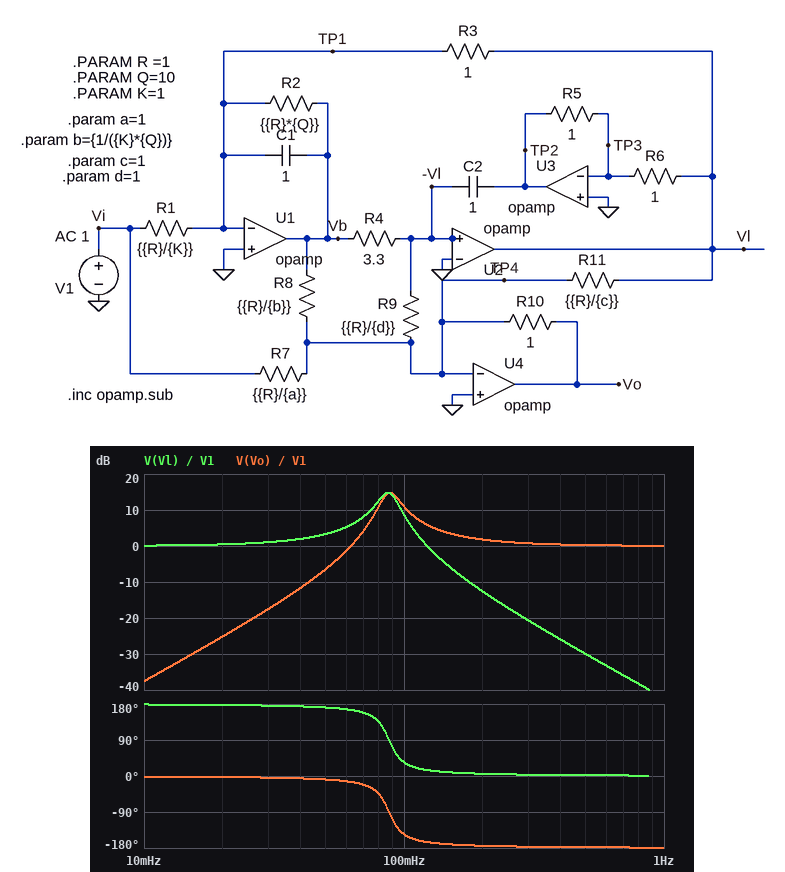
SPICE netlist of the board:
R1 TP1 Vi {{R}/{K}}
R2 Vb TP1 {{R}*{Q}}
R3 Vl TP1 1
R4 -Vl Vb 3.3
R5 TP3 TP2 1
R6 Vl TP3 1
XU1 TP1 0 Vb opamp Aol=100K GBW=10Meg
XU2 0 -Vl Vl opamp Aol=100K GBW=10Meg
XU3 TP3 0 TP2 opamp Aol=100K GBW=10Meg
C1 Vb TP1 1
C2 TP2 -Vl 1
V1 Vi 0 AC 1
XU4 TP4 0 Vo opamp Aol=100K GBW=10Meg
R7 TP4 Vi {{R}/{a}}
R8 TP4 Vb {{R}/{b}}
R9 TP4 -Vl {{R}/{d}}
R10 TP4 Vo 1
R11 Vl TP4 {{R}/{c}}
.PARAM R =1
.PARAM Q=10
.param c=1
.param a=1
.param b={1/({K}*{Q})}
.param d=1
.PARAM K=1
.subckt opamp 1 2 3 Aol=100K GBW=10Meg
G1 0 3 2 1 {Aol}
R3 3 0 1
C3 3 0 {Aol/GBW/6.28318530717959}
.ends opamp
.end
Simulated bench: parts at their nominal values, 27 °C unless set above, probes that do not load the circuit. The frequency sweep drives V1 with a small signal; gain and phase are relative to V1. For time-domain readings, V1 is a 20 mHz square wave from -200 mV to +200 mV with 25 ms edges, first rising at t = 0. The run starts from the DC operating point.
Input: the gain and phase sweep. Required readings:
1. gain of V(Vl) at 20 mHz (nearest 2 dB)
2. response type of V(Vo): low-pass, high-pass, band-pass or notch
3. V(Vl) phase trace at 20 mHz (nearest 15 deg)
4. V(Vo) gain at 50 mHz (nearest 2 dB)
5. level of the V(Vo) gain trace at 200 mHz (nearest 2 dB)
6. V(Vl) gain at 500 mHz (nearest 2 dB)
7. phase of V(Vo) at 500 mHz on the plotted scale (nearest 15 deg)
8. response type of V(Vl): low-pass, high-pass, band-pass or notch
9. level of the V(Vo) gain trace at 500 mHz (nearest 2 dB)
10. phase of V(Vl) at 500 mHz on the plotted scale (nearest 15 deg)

0 dB
high-pass
180 deg
-6 dB
2 dB
-30 dB
-180 deg
low-pass
0 dB
0 deg
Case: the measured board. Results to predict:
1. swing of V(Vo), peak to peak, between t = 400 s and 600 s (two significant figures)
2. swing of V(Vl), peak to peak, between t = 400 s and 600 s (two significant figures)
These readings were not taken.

690 mV
910 mV
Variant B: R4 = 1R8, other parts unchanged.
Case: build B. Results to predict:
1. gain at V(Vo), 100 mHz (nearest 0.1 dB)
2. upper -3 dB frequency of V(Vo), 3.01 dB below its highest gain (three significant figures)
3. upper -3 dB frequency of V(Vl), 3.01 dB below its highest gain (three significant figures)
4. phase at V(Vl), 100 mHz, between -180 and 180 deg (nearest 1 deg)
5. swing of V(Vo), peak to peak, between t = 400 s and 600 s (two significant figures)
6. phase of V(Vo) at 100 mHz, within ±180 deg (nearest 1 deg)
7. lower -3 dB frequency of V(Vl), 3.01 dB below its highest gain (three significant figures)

7.2 dB
128 mHz
126 mHz
159 deg
620 mV
-21 deg
110 mHz
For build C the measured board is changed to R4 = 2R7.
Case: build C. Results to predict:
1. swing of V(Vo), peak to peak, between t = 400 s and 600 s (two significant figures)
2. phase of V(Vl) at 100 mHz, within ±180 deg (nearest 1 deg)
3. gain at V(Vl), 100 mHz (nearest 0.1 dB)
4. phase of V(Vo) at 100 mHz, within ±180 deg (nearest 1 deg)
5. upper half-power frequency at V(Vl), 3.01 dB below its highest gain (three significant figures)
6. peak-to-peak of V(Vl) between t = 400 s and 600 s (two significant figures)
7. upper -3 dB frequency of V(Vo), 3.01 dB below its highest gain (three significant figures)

1.0 V
69 deg
14.8 dB
-111 deg
104 mHz
1.2 V
107 mHz
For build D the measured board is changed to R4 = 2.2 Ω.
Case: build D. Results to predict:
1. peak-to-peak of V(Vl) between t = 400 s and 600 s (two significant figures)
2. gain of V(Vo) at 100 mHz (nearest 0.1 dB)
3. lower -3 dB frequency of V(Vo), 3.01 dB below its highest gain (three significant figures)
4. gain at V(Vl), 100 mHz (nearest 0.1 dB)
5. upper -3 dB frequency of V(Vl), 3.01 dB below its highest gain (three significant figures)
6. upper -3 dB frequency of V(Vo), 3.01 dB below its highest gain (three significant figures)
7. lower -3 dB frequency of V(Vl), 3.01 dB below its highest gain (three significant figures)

1.1 V
13.2 dB
101 mHz
14.4 dB
114 mHz
117 mHz
98.4 mHz
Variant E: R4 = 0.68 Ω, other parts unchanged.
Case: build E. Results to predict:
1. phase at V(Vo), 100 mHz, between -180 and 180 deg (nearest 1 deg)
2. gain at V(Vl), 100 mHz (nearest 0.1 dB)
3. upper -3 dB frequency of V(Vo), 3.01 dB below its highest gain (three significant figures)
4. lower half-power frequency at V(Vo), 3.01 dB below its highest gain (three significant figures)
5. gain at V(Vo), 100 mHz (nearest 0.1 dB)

-3 deg
2.7 dB
202 mHz
186 mHz
-8.7 dB
